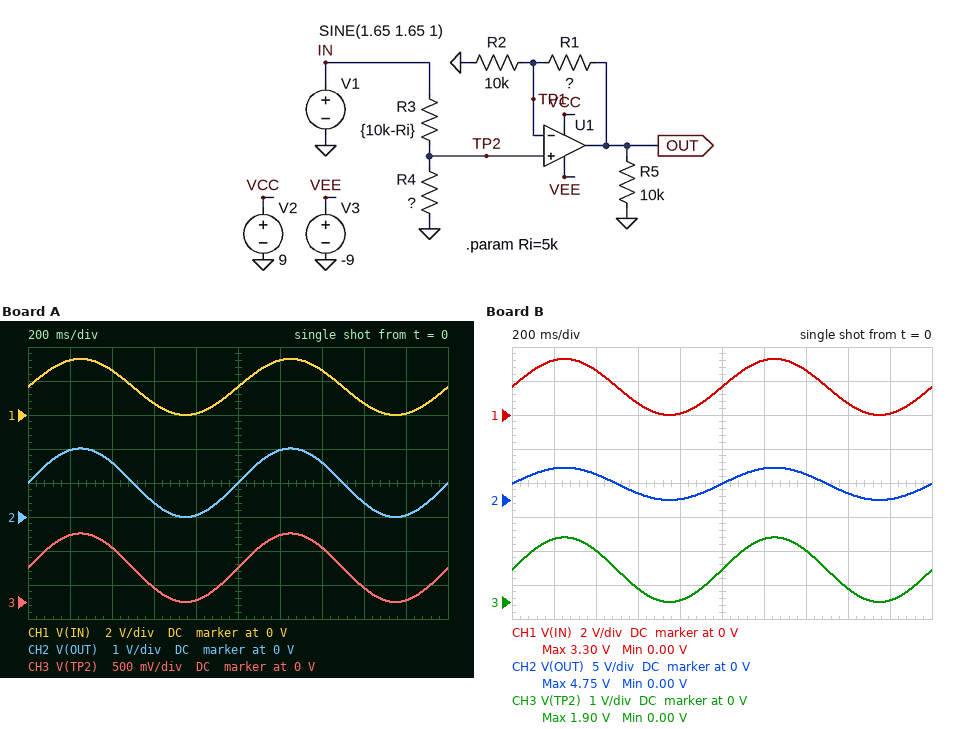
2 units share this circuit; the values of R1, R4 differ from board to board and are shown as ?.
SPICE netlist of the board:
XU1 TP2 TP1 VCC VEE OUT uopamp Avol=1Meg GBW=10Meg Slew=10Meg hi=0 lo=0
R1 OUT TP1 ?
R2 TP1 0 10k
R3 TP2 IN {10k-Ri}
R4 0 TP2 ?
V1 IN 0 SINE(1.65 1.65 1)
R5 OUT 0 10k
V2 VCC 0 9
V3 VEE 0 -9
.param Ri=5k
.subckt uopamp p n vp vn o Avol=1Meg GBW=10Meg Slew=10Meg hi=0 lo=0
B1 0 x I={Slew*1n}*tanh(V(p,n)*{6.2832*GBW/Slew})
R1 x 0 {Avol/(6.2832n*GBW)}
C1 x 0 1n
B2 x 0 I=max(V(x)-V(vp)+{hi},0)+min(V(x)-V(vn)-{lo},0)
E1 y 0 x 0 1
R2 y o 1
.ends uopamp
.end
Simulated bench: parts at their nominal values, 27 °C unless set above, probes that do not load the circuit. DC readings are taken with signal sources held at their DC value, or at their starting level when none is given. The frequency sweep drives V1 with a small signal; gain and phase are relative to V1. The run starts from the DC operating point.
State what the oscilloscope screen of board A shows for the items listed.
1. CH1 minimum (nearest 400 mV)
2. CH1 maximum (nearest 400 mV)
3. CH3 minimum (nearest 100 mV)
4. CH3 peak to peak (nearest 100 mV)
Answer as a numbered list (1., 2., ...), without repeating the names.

1. 0 V
2. 3.2 V
3. 0 V
4. 1.0 V
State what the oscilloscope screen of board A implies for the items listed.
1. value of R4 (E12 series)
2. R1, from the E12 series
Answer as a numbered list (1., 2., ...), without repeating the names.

1. 2.2 kΩ
2. 10 kΩ
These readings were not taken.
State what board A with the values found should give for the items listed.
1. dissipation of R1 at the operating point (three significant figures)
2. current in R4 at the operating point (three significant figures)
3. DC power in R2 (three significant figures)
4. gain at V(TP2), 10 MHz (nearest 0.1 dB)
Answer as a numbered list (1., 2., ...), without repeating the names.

1. 25.4 µW
2. 229 µA
3. 25.4 µW
4. -10.3 dB
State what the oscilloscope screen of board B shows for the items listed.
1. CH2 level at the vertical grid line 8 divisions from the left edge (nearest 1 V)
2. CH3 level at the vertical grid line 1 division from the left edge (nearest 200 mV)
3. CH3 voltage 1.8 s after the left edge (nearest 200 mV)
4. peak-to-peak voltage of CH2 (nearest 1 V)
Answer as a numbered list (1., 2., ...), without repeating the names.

1. 1 V
2. 1.8 V
3. 0 V
4. 5 V
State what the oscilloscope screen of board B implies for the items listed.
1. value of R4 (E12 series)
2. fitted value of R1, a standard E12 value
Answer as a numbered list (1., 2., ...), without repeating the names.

1. 6.8 kΩ
2. 15 kΩ
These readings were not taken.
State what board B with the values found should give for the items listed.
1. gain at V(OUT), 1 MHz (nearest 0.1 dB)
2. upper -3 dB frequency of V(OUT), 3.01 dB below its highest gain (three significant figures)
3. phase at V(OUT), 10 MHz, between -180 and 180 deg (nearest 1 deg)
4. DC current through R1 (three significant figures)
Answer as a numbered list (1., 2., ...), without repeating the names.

1. 2.9 dB
2. 4.00 MHz
3. -68 deg
4. 95.1 µA
